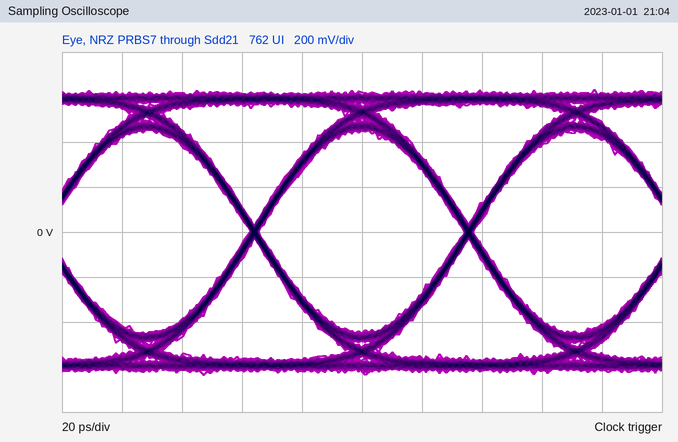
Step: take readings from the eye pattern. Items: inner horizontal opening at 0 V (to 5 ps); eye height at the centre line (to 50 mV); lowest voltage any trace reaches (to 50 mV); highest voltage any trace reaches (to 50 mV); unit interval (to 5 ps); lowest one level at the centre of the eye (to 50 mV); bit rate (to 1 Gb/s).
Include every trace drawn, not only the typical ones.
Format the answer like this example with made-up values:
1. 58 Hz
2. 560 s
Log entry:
1. 70 ps
2. 900 mV
3. -650 mV
4. 650 mV
5. 70 ps
6. 450 mV
7. 14 Gb/s
